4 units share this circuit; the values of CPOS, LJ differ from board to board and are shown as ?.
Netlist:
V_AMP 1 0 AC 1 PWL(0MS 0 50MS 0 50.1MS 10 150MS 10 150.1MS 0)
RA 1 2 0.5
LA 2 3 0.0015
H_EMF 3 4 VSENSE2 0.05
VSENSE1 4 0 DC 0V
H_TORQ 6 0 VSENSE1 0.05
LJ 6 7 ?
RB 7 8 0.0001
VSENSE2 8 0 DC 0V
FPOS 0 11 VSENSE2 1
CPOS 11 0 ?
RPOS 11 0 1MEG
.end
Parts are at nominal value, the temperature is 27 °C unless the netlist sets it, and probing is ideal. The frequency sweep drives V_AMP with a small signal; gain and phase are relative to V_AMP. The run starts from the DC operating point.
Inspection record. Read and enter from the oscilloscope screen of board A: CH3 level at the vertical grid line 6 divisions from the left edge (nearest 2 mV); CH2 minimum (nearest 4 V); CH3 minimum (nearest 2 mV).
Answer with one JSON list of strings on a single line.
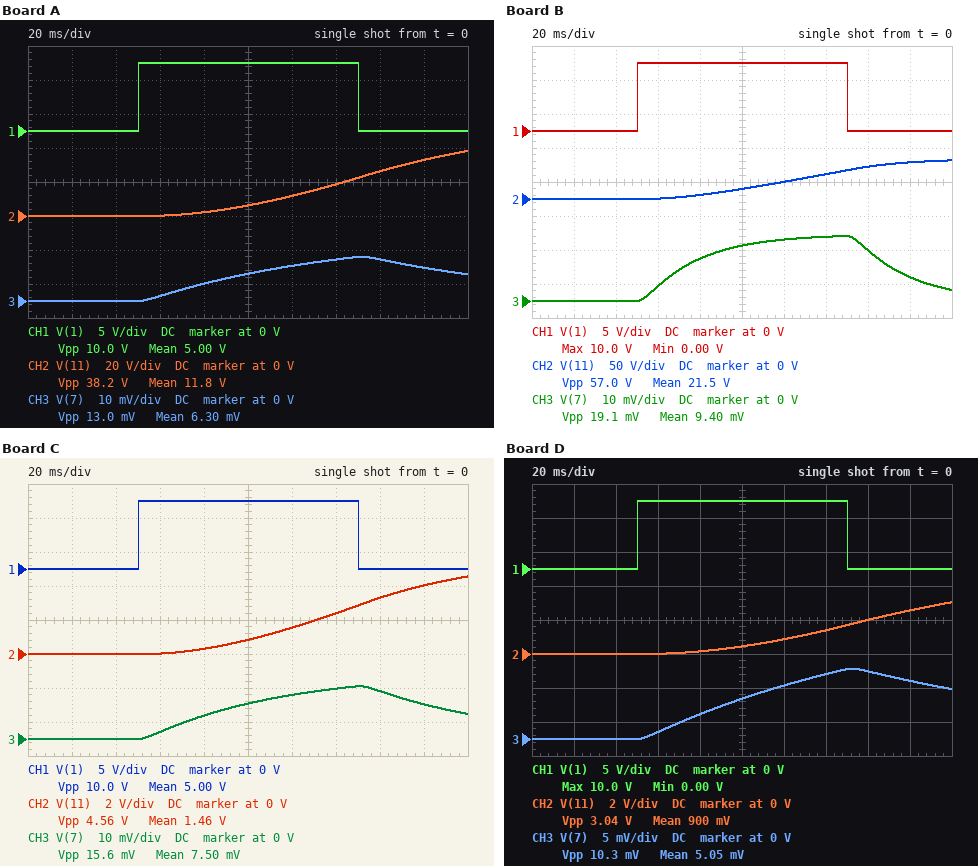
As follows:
["10 mV", "0 V", "0 V"]
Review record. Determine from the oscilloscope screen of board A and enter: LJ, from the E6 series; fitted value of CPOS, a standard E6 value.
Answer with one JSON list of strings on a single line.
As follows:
["470 µH", "330 mF"]
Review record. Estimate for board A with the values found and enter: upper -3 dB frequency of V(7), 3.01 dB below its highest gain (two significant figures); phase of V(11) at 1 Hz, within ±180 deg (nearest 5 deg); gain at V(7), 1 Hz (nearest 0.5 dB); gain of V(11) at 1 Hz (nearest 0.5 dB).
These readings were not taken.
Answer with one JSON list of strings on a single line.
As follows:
["1.8 Hz", "-120 deg", "-55.5 dB", "18.5 dB"]
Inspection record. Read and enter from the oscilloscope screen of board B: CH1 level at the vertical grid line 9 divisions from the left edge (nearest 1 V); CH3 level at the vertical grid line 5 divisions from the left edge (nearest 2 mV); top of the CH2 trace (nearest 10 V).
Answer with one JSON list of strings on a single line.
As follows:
["0 V", "16 mV", "60 V"]
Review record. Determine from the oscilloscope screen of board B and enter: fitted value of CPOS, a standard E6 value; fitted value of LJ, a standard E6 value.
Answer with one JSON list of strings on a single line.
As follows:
["330 mF", "150 µH"]
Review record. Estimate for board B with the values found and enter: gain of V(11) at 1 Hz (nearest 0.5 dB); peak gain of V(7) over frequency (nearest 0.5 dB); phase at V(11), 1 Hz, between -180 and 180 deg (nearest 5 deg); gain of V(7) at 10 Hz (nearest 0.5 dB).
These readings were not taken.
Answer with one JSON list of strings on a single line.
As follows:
["19.5 dB", "-54.0 dB", "-100 deg", "-60.0 dB"]
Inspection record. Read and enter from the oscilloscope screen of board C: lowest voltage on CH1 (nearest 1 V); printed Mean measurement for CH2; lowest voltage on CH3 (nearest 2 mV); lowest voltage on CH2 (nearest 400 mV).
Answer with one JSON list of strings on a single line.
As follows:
["0 V", "1.46 V", "0 V", "0 V"]
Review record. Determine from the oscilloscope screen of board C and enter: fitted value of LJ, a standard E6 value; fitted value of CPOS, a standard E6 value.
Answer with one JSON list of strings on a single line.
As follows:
["330 µH", "3.3 F"]
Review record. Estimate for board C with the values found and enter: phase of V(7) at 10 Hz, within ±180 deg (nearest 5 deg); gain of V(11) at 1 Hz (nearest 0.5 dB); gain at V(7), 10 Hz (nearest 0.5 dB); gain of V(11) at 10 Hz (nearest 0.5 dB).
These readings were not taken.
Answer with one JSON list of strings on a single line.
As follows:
["-85 deg", "-1.0 dB", "-66.5 dB", "-32.5 dB"]
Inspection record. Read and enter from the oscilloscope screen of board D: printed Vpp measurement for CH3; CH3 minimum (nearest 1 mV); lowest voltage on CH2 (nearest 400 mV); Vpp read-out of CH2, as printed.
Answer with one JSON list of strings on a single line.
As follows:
["10.3 mV", "0 V", "0 V", "3.04 V"]
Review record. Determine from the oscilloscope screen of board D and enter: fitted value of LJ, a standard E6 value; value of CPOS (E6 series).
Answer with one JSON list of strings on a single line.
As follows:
["680 µH", "3.3 F"]
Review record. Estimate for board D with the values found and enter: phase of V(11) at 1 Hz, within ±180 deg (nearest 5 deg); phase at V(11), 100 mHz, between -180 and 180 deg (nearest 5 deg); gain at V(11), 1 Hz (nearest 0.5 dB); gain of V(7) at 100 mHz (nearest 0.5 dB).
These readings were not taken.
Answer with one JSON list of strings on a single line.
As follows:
["-130 deg", "-95 deg", "-2.5 dB", "-54.0 dB"]
